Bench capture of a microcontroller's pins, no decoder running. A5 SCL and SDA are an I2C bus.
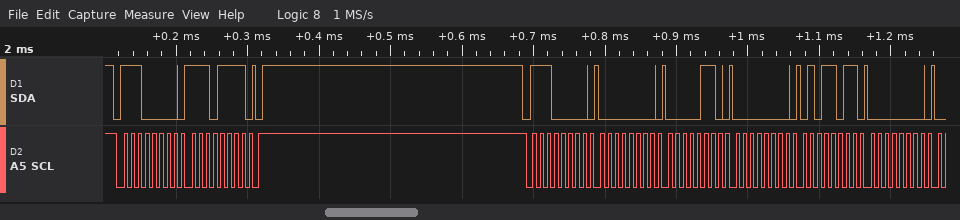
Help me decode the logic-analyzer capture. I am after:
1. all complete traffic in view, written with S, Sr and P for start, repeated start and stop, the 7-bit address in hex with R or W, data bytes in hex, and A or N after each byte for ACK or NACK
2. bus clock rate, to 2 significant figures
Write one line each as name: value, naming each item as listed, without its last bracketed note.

all complete traffic in view, written with S, Sr and P for start, repeated start and stop, the 7-bit address in hex with R or W, data bytes in hex, and A or N after each byte for ACK or NACK: S 70W A EF A P S 70W A 00 A 06 A 00 A 5B A 00 A
bus clock rate, to 2 significant figures: 100 kHz
